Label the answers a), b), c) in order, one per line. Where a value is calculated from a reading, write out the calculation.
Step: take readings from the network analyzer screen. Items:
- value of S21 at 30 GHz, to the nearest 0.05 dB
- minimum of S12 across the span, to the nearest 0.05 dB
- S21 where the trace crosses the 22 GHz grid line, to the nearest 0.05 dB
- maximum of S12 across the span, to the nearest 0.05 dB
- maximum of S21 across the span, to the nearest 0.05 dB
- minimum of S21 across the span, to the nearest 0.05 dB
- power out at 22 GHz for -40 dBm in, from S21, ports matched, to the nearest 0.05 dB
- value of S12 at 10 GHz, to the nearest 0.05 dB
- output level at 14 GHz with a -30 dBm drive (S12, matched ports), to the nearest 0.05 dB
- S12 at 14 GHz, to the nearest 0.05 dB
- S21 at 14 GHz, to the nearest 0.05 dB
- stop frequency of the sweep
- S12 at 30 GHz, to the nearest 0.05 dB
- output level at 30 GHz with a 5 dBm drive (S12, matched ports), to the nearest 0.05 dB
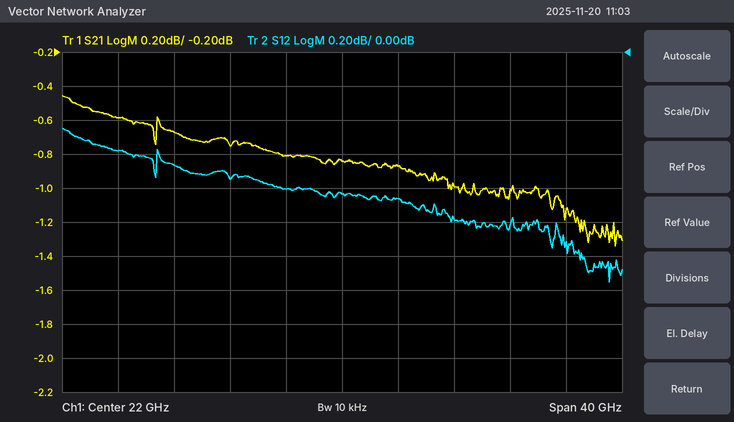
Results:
a) -1.00 dB
b) -1.35 dB
c) -0.85 dB
d) -0.45 dB
e) -0.45 dB
f) -1.35 dB
g) -40 dBm + (-0.85 dB) = -40.85 dBm
h) -0.65 dB
i) -30 dBm + (-0.75 dB) = -30.75 dBm
j) -0.75 dB
k) -0.75 dB
l) 42 GHz
m) -1.00 dB
n) 5 dBm + (-1.00 dB) = 4.00 dBm
